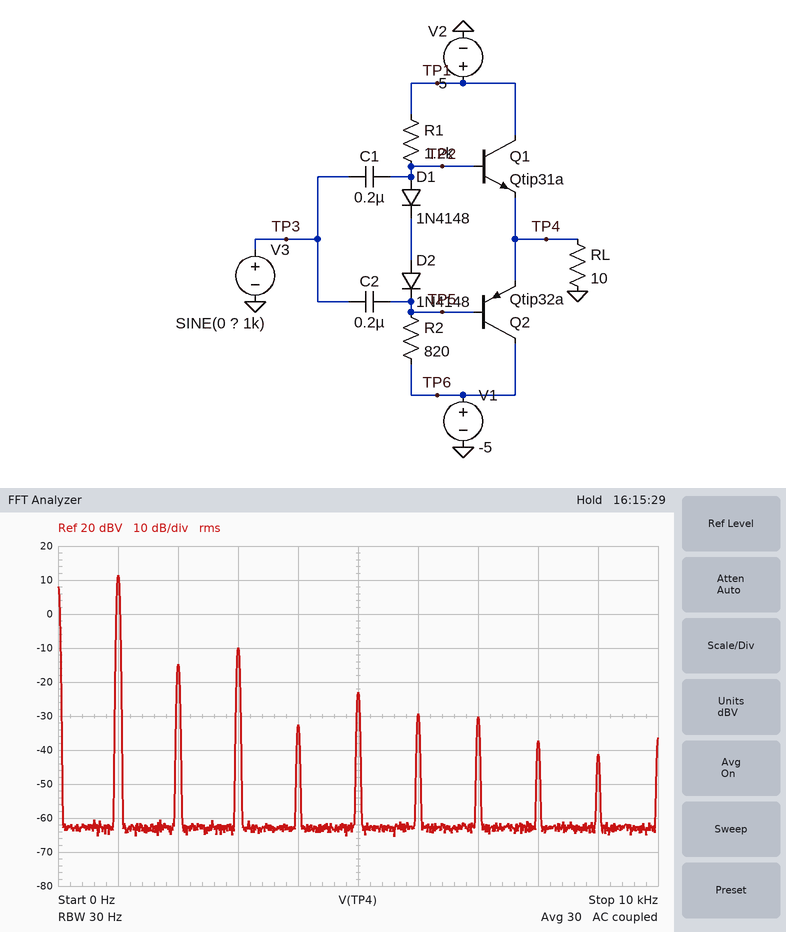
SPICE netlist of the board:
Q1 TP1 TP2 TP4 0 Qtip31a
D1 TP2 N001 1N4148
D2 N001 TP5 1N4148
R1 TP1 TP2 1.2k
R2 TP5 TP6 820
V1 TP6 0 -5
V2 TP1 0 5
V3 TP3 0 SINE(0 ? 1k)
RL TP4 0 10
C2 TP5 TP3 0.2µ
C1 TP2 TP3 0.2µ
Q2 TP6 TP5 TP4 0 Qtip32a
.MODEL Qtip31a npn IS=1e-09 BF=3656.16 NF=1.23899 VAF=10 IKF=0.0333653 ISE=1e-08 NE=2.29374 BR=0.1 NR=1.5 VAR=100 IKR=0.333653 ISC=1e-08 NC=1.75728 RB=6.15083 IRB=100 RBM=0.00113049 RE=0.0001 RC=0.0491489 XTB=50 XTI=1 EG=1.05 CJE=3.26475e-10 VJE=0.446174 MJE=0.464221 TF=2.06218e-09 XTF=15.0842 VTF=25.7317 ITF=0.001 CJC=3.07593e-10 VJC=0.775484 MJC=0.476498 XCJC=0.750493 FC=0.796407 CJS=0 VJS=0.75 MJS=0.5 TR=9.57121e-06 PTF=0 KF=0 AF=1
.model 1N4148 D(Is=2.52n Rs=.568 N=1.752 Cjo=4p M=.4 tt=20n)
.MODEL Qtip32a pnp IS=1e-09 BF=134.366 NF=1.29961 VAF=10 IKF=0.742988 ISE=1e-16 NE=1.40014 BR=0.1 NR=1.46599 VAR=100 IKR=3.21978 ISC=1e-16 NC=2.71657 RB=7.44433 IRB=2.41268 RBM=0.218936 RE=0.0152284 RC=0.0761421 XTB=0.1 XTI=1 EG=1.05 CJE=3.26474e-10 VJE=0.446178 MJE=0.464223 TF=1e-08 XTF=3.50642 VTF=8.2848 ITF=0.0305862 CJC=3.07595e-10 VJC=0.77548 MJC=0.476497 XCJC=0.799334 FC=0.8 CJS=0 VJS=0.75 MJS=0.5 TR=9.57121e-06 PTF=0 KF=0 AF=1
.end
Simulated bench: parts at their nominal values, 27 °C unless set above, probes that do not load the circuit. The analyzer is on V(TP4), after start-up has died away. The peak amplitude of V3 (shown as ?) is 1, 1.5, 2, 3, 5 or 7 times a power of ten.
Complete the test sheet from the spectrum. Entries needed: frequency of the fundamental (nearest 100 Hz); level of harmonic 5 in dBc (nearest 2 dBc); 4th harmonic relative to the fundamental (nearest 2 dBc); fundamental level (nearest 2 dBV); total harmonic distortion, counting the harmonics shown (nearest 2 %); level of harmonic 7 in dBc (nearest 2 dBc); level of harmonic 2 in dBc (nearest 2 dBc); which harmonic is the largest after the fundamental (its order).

1.0 kHz
-34 dBc
-44 dBc
12 dBV
10 %
-42 dBc
-26 dBc
3
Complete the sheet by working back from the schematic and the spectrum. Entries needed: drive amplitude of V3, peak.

10 V
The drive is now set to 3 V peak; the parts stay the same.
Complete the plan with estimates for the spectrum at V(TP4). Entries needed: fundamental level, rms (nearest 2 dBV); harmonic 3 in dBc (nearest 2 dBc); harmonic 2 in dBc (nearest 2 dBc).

2 dBV
-56 dBc
-46 dBc
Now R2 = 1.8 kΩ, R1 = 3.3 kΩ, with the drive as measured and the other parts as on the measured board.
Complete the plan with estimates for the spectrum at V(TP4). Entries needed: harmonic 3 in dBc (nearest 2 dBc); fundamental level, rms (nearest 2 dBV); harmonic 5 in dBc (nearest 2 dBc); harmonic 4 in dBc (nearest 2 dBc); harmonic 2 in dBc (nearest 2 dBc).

-24 dBc
12 dBV
-28 dBc
-22 dBc
-20 dBc
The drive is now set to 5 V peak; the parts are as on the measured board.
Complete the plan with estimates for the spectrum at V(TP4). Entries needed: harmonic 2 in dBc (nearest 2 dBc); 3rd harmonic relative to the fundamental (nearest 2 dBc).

-40 dBc
-46 dBc
